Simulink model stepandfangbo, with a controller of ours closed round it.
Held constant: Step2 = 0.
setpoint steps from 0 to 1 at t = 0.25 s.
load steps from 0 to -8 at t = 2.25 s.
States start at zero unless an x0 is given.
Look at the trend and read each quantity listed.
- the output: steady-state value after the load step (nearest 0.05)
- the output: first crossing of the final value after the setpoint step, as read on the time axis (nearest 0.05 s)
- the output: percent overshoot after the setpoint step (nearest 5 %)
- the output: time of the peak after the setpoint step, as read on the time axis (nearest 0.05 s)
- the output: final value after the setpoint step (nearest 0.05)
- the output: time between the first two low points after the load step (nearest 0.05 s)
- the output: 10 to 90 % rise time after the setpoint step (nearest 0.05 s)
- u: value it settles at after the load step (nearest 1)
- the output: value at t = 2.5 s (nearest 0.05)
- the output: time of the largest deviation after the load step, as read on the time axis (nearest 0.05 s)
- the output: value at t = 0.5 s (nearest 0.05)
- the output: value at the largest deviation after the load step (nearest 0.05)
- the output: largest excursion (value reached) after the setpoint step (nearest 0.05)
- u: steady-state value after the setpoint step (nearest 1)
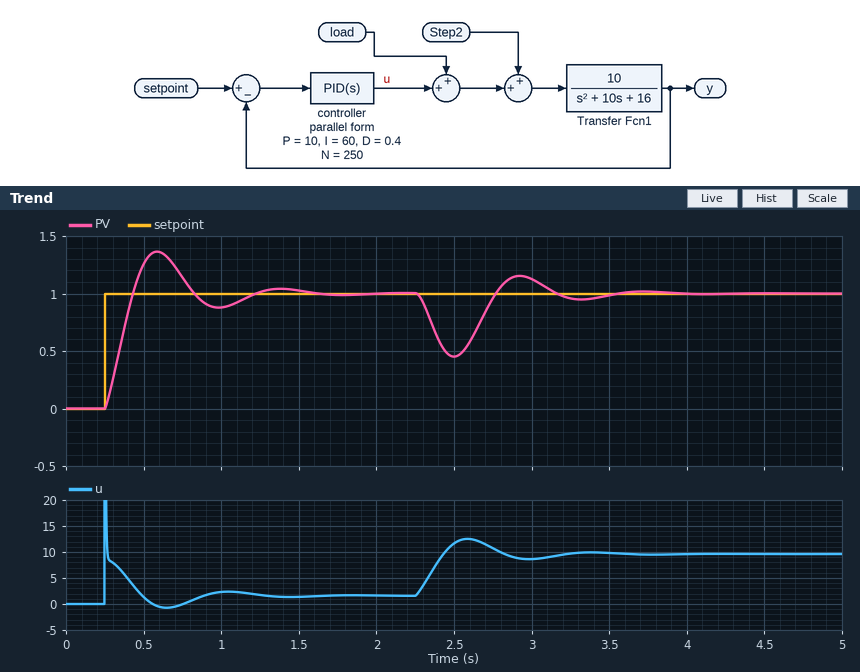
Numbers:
1.00
0.45 s
35 %
0.60 s
1.00
0.80 s
0.15 s
10
0.45
2.50 s
1.25
0.45
1.35
2
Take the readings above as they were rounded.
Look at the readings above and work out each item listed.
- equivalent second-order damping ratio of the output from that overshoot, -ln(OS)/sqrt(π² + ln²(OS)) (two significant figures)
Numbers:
0.32
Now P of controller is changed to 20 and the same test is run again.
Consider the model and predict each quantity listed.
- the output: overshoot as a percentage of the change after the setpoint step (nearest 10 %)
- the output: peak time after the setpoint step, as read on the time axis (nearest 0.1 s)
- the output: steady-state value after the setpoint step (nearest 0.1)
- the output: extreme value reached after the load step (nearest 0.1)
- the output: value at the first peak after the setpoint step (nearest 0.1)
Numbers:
30 %
0.5 s
1.0
0.6
1.3
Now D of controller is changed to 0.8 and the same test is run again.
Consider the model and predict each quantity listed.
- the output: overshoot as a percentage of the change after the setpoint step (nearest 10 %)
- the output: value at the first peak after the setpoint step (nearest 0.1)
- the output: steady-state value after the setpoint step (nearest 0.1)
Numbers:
20 %
1.2
1.0
